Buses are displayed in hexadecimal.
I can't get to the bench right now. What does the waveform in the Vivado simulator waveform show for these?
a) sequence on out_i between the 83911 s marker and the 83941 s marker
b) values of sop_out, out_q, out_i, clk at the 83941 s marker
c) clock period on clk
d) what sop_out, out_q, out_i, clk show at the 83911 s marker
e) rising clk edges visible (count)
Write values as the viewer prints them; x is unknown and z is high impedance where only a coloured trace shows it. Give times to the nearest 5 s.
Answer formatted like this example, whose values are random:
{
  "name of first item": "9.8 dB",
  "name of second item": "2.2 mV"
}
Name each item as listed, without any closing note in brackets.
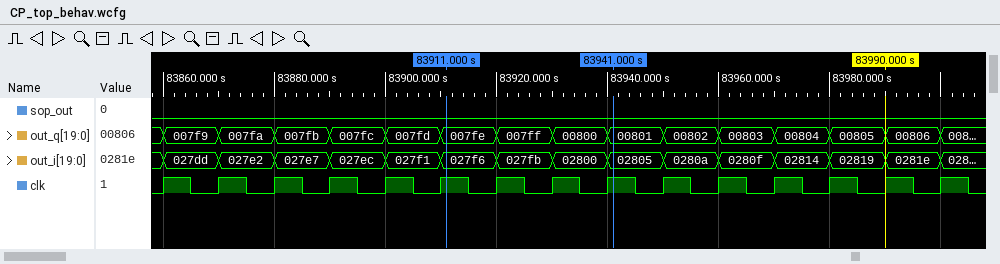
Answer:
{
  "sequence on out_i between the 83911 s marker and the 83941 s marker": "027f6, 027fb, 02800, 02805",
  "values of sop_out, out_q, out_i, clk at the 83941 s marker": "sop_out=0, out_q=00801, out_i=02805, clk=1",
  "clock period on clk": "10 s",
  "what sop_out, out_q, out_i, clk show at the 83911 s marker": "sop_out=0, out_q=007fe, out_i=027f6, clk=1",
  "rising clk edges visible": "15"
}
